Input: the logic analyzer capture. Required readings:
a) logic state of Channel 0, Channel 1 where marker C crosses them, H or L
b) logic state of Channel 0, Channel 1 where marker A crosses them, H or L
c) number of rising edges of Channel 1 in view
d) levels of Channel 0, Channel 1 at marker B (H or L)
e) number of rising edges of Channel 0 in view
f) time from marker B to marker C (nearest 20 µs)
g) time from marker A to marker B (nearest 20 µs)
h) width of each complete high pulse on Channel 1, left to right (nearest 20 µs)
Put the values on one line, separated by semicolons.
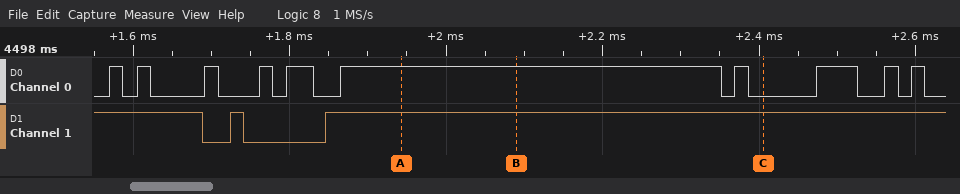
Channel 0=L, Channel 1=H; Channel 0=H, Channel 1=H; 2; Channel 0=H, Channel 1=H; 10; 320 µs; 140 µs; 20 µs
